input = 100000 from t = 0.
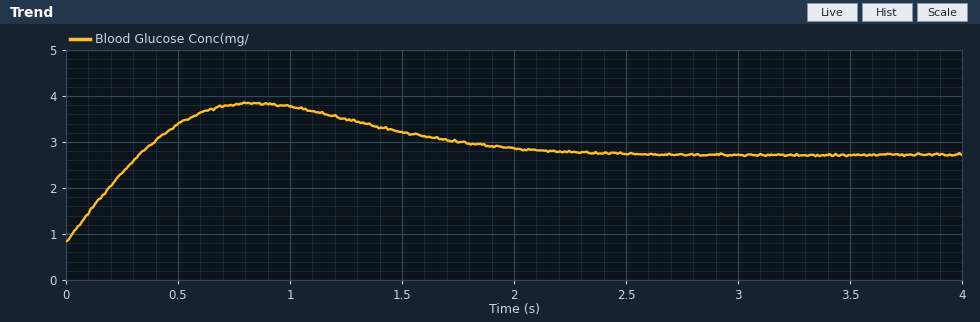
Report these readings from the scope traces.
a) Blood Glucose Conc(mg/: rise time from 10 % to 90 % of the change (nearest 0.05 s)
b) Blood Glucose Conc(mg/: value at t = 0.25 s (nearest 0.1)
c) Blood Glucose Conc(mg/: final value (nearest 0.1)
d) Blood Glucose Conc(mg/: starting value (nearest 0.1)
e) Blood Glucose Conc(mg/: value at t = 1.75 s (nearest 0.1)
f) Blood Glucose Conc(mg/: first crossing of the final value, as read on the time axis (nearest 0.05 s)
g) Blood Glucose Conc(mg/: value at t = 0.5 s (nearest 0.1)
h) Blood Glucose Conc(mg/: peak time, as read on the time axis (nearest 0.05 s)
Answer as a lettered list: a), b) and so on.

a) 0.25 s
b) 2.3
c) 2.7
d) 0.8
e) 3.0
f) 0.35 s
g) 3.4
h) 0.85 s
